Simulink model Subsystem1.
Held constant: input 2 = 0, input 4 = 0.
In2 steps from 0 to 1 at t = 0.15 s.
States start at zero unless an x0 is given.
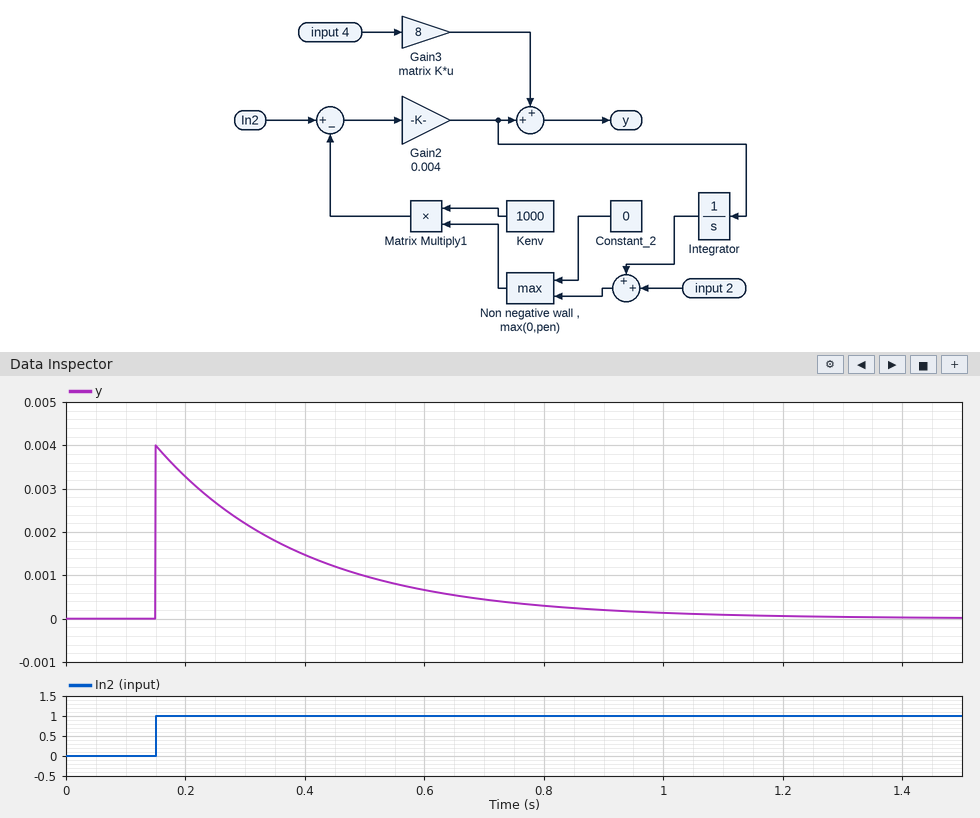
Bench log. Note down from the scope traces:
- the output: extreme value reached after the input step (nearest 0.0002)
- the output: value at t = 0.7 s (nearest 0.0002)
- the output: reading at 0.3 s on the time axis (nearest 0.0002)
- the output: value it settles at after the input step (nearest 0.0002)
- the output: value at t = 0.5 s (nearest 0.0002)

0.0040
0.0004
0.0022
0.0000
0.0010
